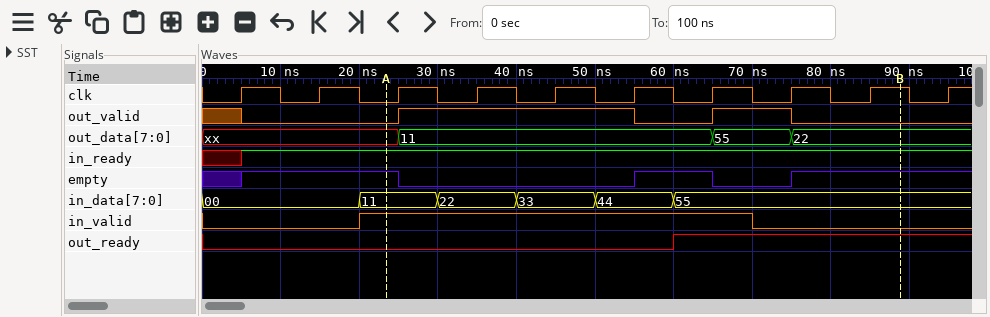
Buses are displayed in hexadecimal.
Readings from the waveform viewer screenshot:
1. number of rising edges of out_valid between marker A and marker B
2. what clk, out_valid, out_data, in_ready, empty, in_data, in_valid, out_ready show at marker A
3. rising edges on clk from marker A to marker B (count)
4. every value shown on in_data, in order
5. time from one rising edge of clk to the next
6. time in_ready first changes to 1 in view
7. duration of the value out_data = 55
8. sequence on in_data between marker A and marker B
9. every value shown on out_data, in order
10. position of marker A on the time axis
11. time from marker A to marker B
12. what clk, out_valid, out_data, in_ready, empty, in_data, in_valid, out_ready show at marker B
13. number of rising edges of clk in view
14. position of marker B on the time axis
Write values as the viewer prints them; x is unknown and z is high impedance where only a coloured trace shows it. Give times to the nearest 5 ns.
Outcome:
2
clk=0, out_valid=0, out_data=xx, in_ready=1, empty=1, in_data=11, in_valid=1, out_ready=0
7
00, 11, 22, 33, 44, 55
10 ns
5 ns
10 ns
11, 22, 33, 44, 55
xx, 11, 55, 22
25 ns
65 ns
clk=1, out_valid=0, out_data=22, in_ready=1, empty=1, in_data=55, in_valid=0, out_ready=1
10
90 ns
